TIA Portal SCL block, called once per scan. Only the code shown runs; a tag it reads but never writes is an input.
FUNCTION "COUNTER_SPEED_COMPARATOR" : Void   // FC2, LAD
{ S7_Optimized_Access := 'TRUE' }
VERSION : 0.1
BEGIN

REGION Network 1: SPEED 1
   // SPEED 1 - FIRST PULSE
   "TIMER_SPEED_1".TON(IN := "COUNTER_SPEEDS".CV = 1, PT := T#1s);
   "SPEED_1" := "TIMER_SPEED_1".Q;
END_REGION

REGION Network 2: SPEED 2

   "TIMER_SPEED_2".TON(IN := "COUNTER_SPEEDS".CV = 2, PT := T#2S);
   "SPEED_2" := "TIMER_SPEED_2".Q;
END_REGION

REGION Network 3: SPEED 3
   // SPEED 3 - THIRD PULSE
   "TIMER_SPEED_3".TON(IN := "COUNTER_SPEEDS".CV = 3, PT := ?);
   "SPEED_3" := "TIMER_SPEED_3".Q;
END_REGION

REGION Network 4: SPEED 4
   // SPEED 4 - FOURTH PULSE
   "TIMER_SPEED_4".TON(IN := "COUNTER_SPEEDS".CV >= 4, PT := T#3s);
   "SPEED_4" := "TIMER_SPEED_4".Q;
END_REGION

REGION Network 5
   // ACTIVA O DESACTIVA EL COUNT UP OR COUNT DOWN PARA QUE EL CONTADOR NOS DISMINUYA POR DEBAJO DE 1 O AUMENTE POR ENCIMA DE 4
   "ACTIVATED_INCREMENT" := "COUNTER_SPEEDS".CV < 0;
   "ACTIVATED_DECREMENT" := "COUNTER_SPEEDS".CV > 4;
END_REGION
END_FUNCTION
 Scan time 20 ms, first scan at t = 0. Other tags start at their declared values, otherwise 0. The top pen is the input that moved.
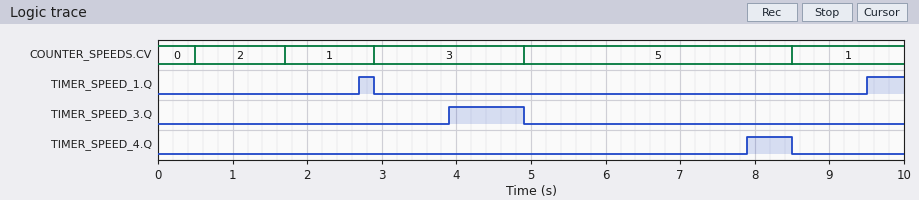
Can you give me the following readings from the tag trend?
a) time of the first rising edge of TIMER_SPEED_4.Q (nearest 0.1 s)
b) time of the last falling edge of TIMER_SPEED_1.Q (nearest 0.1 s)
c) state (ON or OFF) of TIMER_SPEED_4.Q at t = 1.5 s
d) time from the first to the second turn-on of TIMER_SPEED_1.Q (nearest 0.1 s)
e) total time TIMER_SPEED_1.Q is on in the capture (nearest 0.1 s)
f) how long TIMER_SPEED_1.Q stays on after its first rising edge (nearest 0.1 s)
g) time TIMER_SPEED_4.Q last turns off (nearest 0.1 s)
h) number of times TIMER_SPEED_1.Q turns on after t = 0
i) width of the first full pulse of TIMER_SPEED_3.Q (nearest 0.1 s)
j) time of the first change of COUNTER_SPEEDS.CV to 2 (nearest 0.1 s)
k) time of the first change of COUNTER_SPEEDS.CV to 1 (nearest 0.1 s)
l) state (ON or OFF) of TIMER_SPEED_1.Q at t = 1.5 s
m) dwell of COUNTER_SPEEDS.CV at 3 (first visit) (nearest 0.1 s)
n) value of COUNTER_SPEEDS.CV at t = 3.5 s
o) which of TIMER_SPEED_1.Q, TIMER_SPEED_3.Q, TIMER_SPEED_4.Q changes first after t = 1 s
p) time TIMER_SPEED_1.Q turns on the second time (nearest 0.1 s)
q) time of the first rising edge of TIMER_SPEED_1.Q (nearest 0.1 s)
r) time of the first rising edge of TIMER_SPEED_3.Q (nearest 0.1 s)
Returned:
7.9 s
2.9 s
OFF
6.8 s
0.7 s
0.2 s
8.5 s
2
1.0 s
0.5 s
1.7 s
OFF
2.0 s
3
TIMER_SPEED_1.Q
9.5 s
2.7 s
3.9 s
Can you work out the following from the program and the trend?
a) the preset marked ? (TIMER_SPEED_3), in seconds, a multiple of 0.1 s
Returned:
1.0 s
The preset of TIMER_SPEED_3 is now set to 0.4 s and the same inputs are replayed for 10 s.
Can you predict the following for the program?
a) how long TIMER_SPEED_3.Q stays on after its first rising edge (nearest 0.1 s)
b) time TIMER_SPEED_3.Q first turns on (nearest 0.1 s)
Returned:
1.6 s
3.3 s
